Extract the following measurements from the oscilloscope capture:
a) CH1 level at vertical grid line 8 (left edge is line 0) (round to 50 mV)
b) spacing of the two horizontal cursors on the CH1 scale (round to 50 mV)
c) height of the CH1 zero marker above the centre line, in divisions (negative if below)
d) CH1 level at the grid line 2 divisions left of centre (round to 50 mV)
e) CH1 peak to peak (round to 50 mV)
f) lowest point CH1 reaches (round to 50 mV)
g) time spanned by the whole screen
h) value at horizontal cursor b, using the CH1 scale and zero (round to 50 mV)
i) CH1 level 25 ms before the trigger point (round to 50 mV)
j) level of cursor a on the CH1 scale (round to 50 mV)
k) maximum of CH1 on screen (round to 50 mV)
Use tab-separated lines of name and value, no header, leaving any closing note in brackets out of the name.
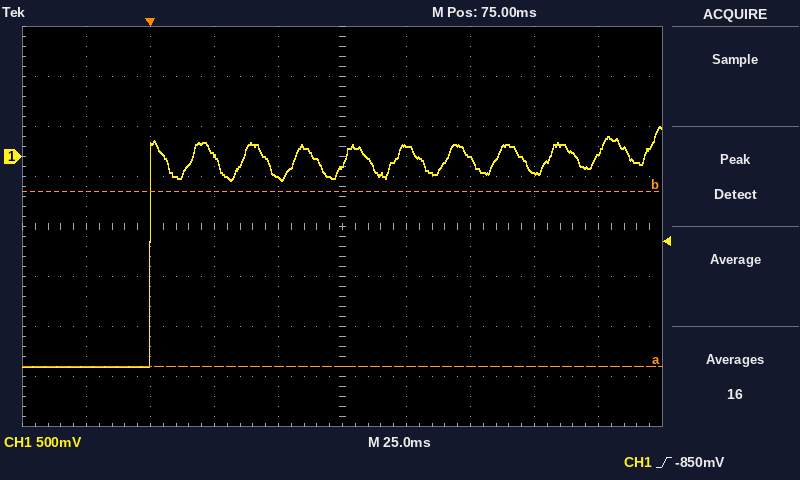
CH1 level at vertical grid line 8 (left edge is line 0)	-150 mV
spacing of the two horizontal cursors on the CH1 scale	1.75 V
height of the CH1 zero marker above the centre line, in divisions	+1.4 div
CH1 level at the grid line 2 divisions left of centre	0 mV
CH1 peak to peak	2.40 V
lowest point CH1 reaches	-2.10 V
time spanned by the whole screen	250 ms
value at horizontal cursor b, using the CH1 scale and zero	-350 mV
CH1 level 25 ms before the trigger point	-2.10 V
level of cursor a on the CH1 scale	-2.10 V
maximum of CH1 on screen	300 mV
